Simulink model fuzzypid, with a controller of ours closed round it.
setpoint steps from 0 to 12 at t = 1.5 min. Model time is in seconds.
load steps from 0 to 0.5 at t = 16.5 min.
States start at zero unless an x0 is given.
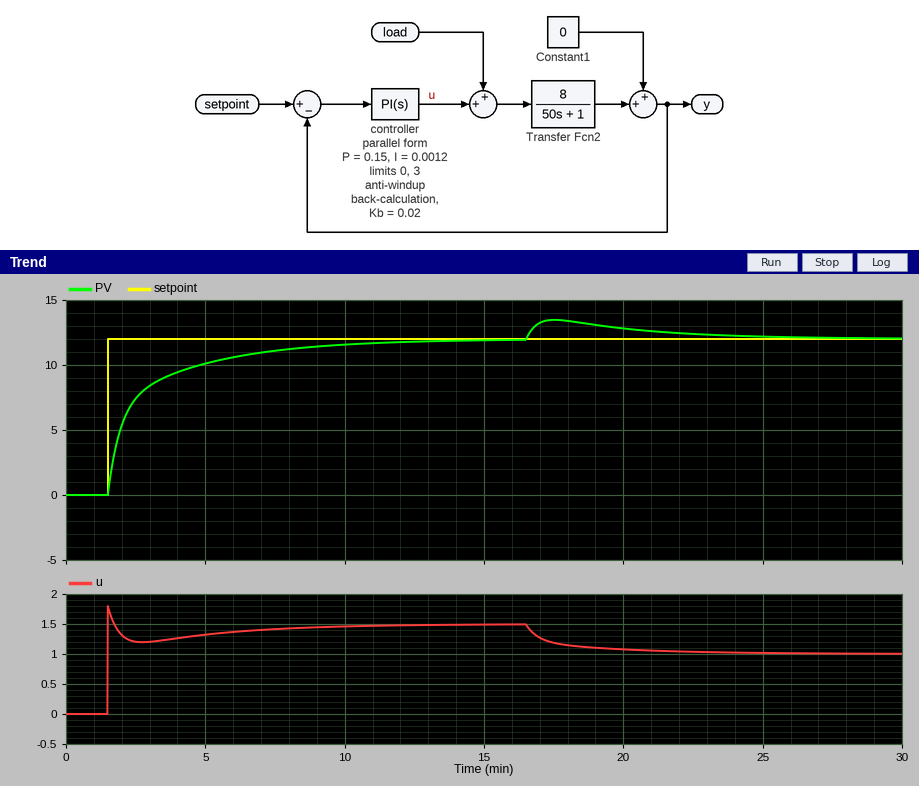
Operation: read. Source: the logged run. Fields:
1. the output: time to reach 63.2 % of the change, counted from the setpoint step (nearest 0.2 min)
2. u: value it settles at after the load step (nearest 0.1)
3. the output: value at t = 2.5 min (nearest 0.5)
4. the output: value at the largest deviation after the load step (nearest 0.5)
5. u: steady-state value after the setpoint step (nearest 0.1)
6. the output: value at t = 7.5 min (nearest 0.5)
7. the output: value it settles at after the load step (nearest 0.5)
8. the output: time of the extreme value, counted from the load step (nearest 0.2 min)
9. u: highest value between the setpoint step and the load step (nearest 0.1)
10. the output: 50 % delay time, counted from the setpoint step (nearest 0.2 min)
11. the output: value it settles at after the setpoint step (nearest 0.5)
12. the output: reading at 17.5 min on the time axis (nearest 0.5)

1.0 min
1.0
7.5
13.5
1.5
11.0
12.0
1.0 min
1.8
0.6 min
12.0
13.5
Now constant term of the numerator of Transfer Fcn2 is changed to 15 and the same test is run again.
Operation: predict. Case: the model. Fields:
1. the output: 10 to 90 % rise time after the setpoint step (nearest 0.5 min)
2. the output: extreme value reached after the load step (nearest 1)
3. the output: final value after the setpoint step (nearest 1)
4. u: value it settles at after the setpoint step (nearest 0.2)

2.5 min
14
12
0.8
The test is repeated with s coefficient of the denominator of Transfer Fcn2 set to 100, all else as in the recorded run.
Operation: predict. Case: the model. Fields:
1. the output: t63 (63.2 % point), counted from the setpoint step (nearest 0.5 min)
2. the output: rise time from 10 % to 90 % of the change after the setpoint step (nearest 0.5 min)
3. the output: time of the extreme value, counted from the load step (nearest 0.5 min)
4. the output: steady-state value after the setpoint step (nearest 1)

1.5 min
4.0 min
1.5 min
12
